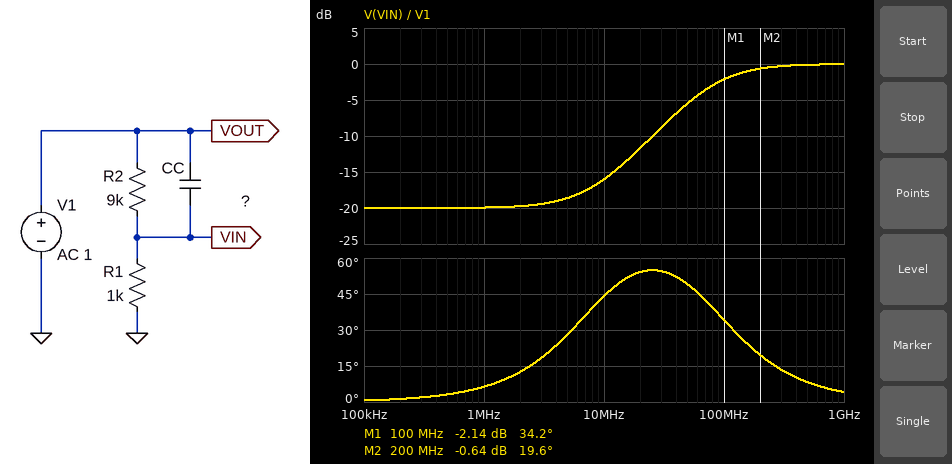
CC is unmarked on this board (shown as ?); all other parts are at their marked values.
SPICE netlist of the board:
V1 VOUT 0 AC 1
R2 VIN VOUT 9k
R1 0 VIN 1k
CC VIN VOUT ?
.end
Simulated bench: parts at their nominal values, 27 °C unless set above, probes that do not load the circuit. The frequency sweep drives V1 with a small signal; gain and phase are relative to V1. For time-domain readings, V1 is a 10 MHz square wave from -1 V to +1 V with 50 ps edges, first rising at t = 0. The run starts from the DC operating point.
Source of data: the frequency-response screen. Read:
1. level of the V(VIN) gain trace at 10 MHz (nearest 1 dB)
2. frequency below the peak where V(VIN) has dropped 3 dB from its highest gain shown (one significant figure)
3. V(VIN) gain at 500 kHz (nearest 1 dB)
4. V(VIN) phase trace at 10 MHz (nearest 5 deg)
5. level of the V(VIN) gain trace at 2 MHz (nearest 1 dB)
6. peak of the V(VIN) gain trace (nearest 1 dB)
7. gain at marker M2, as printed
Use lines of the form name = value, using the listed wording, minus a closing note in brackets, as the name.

level of the V(VIN) gain trace at 10 MHz = -16 dB
frequency below the peak where V(VIN) has dropped 3 dB from its highest gain shown = 80 MHz
V(VIN) gain at 500 kHz = -20 dB
V(VIN) phase trace at 10 MHz = 45 deg
level of the V(VIN) gain trace at 2 MHz = -20 dB
peak of the V(VIN) gain trace = 0 dB
gain at marker M2, as printed = -0.64 dB
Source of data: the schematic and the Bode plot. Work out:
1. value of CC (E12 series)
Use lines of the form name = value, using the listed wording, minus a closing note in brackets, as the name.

value of CC = 2.2 pF
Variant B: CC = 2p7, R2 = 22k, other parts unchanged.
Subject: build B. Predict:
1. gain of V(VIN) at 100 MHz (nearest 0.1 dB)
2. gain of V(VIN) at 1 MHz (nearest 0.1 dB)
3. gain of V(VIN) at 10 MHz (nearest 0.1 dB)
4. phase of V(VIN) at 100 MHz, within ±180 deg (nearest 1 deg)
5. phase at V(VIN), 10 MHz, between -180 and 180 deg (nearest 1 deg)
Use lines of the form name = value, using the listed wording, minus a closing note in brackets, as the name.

gain of V(VIN) at 100 MHz = -1.4 dB
gain of V(VIN) at 1 MHz = -26.7 dB
gain of V(VIN) at 10 MHz = -15.6 dB
phase of V(VIN) at 100 MHz, within ±180 deg = 30 deg
phase at V(VIN), 10 MHz, between -180 and 180 deg = 66 deg
